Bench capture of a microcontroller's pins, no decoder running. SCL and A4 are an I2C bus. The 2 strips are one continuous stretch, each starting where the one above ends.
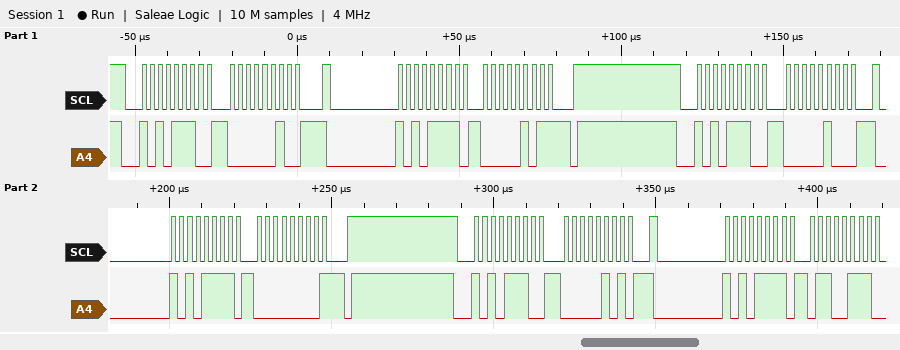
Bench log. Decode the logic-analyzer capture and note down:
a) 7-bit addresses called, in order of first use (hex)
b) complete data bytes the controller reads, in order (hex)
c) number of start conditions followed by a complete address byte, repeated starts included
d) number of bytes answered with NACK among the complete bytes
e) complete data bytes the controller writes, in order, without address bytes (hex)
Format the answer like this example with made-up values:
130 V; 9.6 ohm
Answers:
0x57; 05 00 67; 6; 2; 02 04 05
